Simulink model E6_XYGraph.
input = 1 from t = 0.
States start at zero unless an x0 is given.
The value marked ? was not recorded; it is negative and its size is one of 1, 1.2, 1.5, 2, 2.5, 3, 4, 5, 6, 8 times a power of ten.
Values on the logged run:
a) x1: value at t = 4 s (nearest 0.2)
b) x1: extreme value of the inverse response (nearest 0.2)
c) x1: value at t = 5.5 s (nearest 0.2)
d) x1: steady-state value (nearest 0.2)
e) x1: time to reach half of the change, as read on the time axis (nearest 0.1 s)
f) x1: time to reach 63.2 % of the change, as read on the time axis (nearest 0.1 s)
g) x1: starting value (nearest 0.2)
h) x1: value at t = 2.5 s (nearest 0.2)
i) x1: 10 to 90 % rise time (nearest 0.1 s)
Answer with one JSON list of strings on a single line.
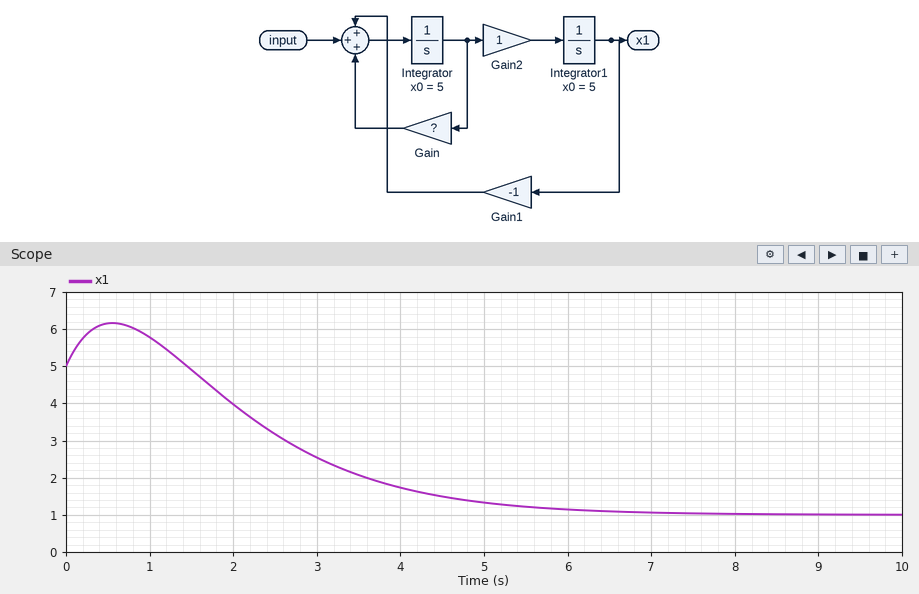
["1.8", "6.2", "1.2", "1.0", "2.6 s", "3.1 s", "5.0", "3.2", "3.1 s"]
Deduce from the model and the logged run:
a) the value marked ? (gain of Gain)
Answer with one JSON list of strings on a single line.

["-2"]
